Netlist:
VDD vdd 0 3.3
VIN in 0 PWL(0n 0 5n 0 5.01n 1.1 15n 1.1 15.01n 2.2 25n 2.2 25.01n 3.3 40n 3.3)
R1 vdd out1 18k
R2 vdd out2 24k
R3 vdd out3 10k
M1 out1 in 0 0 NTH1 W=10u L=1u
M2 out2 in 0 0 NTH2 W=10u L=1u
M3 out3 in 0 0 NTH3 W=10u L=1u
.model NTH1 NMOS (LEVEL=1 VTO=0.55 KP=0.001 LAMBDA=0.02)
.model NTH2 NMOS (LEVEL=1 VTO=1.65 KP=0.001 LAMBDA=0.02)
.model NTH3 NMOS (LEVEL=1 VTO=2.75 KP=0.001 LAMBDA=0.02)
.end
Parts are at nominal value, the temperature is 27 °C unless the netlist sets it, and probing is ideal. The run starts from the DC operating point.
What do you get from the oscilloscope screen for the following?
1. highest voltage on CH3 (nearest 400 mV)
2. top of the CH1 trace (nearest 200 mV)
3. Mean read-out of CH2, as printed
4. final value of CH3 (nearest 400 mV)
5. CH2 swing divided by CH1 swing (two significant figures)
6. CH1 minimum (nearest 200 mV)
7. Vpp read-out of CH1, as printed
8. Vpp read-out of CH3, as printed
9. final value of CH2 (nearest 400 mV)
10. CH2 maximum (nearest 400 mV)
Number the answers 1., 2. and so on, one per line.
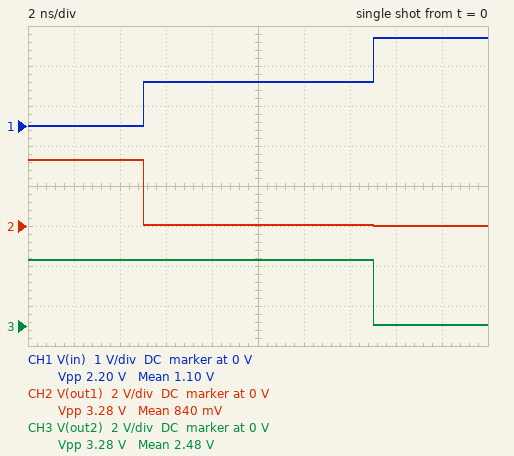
1. 3.2 V
2. 2.2 V
3. 840 mV
4. 0 V
5. 1.5
6. 0 V
7. 2.20 V
8. 3.28 V
9. 0 V
10. 3.2 V
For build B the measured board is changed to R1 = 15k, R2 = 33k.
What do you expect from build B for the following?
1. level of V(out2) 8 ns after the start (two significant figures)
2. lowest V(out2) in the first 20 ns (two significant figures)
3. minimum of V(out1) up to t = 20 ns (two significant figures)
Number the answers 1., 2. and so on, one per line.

1. 3.3 V
2. 18 mV
3. 13 mV
